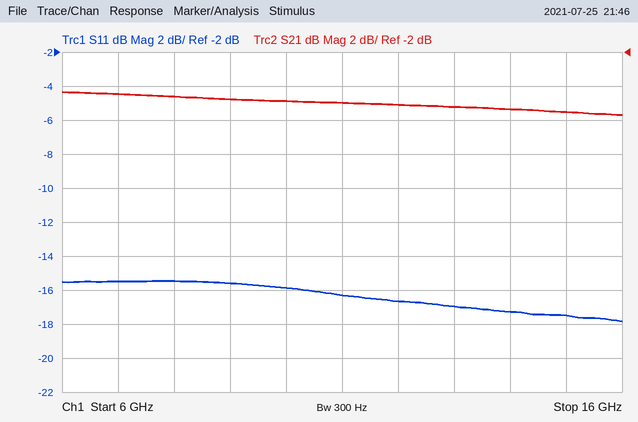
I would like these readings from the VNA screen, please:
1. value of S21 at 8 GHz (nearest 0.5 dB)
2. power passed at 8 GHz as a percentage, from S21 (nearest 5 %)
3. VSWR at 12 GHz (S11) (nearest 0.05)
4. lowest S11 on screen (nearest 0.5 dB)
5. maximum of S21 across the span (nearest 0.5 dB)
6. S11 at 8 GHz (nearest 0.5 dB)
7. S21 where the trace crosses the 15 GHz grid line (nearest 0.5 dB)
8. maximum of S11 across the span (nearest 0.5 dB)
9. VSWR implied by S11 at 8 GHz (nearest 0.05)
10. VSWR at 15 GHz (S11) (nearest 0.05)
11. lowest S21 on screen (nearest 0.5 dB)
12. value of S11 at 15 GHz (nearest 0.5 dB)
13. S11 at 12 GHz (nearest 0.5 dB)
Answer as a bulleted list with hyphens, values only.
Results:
- -4.5 dB
- 35 %
- 1.35
- -18.0 dB
- -4.5 dB
- -15.5 dB
- -5.5 dB
- -15.5 dB
- 1.40
- 1.30
- -5.5 dB
- -17.5 dB
- -16.5 dB
